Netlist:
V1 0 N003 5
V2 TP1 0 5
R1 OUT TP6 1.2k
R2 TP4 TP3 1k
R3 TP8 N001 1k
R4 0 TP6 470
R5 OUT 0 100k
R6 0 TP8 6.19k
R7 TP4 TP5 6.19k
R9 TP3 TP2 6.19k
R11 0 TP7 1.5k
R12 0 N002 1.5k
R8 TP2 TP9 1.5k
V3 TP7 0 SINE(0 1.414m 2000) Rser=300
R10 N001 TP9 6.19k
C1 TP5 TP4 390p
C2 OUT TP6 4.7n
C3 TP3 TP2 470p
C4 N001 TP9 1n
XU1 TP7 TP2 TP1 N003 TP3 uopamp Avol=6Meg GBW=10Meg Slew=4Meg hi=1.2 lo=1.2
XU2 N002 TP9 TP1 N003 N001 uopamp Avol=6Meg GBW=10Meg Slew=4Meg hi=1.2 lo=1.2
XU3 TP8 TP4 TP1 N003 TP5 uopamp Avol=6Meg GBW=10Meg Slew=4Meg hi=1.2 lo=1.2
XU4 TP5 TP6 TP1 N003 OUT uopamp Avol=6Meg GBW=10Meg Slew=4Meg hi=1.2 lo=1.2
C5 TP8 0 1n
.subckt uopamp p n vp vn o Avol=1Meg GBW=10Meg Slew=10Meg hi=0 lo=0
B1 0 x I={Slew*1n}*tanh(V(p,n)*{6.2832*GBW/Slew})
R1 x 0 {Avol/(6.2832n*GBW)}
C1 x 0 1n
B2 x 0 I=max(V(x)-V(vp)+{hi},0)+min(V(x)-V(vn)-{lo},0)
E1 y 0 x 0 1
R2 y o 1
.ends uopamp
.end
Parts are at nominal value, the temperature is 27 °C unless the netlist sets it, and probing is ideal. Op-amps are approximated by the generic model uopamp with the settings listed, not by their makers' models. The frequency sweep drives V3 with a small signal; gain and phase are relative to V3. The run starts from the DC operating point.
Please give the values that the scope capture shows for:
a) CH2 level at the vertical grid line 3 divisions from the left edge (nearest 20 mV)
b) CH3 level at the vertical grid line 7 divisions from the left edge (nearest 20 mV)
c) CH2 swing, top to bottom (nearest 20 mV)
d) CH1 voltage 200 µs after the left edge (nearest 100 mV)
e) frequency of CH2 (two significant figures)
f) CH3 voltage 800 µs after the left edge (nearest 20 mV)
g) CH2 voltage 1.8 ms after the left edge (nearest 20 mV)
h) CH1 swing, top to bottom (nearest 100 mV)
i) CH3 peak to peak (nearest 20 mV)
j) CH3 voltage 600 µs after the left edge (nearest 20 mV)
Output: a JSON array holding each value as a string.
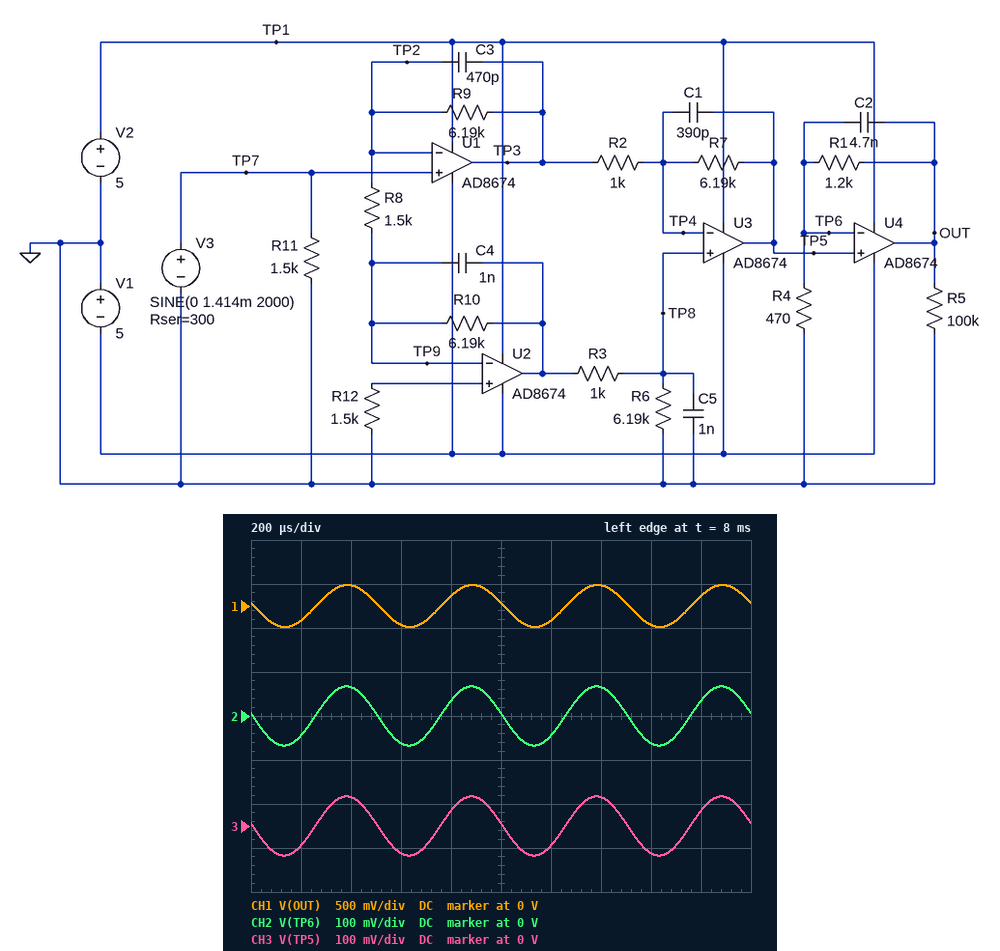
["-60 mV", "60 mV", "140 mV", "-200 mV", "2.0 kHz", "40 mV", "40 mV", "500 mV", "140 mV", "-60 mV"]
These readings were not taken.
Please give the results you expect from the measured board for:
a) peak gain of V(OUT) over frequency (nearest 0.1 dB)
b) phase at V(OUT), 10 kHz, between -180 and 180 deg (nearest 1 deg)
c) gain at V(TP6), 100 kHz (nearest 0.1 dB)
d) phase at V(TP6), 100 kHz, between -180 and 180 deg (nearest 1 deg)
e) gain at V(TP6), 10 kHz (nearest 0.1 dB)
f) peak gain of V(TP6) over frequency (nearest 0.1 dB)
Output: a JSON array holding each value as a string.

["44.6 dB", "142 deg", "18.8 dB", "66 deg", "33.0 dB", "33.6 dB"]
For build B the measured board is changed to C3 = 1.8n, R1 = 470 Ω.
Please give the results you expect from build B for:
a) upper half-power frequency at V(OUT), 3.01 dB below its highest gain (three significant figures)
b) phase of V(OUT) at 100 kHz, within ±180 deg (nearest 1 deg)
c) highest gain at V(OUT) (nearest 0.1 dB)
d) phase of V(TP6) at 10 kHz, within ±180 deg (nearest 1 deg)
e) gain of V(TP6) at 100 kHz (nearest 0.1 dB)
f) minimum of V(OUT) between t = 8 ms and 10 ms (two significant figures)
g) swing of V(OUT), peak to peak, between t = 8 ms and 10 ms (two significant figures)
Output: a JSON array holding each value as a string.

["16.3 kHz", "46 deg", "39.6 dB", "145 deg", "13.9 dB", "-130 mV", "270 mV"]
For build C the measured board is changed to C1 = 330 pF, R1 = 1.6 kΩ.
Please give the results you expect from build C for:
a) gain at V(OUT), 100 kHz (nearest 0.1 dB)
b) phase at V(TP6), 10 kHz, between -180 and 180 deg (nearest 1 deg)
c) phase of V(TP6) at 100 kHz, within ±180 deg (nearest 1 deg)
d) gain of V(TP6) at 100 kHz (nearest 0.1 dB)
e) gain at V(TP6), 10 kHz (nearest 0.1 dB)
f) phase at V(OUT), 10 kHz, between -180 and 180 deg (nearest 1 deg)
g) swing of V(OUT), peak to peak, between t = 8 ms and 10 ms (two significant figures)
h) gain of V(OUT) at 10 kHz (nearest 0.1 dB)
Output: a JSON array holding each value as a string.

["22.2 dB", "157 deg", "70 deg", "19.7 dB", "33.0 dB", "138 deg", "590 mV", "45.1 dB"]
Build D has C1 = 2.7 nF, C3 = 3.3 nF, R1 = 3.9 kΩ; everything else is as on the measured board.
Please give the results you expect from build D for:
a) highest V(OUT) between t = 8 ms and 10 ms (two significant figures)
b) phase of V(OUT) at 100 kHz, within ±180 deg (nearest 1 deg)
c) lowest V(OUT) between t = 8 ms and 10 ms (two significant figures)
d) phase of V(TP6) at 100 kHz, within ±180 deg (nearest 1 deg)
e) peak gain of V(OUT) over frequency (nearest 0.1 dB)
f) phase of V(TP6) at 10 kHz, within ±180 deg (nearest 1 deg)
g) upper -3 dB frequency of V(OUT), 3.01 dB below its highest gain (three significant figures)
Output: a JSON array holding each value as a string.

["590 mV", "23 deg", "-590 mV", "57 deg", "52.9 dB", "107 deg", "4.78 kHz"]
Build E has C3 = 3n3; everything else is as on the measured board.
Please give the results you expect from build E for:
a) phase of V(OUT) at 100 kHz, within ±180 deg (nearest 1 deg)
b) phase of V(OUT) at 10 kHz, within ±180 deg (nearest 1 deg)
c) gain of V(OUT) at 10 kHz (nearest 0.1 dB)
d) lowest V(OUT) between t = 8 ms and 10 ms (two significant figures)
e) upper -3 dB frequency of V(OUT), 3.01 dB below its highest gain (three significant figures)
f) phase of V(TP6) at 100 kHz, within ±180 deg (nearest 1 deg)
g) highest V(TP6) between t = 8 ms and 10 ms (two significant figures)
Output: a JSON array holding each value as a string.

["40 deg", "127 deg", "41.6 dB", "-230 mV", "10.0 kHz", "69 deg", "66 mV"]
